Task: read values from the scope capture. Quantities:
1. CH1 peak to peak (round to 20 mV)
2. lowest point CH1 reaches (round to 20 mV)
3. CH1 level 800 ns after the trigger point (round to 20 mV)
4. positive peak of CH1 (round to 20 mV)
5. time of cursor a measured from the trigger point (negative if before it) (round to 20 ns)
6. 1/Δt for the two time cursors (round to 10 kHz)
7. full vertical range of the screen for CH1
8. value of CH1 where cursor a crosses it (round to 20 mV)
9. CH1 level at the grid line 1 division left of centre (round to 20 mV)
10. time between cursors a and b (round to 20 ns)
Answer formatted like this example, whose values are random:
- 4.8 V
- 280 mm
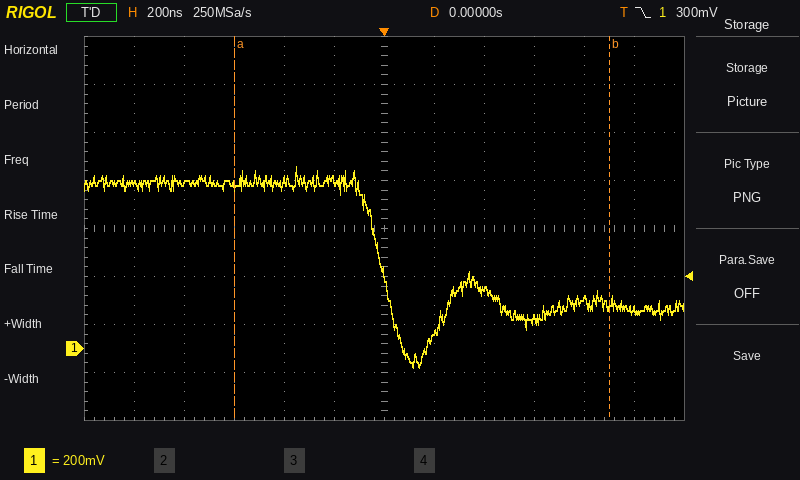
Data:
- 840 mV
- -80 mV
- 200 mV
- 760 mV
- -600 ns
- 670 kHz
- 1.6 V
- 680 mV
- 700 mV
- 1.50 µs
